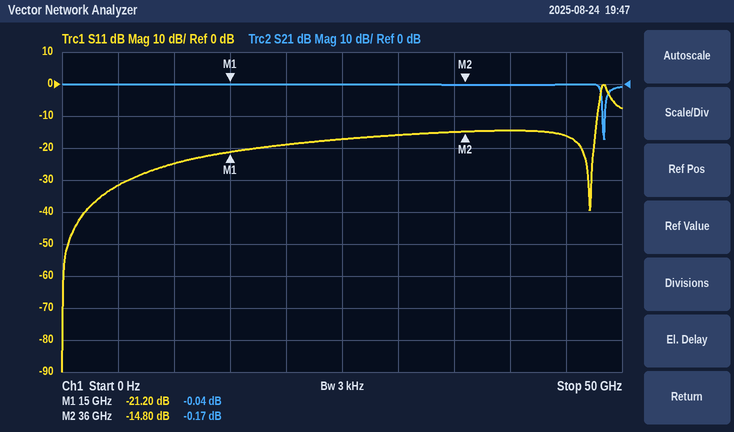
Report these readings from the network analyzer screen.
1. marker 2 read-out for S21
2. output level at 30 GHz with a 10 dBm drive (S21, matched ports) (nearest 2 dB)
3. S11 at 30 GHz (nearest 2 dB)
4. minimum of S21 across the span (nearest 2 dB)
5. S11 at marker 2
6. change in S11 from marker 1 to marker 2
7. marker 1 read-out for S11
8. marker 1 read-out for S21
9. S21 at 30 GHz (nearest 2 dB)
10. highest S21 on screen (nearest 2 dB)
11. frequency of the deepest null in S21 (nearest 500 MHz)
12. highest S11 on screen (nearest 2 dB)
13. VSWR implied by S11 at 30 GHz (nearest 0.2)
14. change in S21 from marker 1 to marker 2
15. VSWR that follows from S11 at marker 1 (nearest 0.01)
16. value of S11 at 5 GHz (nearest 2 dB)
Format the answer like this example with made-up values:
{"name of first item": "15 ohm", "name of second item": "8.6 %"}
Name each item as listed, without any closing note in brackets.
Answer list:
{"marker 2 read-out for S21": "-0.17 dB", "output level at 30 GHz with a 10 dBm drive (S21, matched ports)": "10 dBm", "S11 at 30 GHz": "-16 dB", "minimum of S21 across the span": "-18 dB", "S11 at marker 2": "-14.80 dB", "change in S11 from marker 1 to marker 2": "6.40 dB", "marker 1 read-out for S11": "-21.20 dB", "marker 1 read-out for S21": "-0.04 dB", "S21 at 30 GHz": "0 dB", "highest S21 on screen": "0 dB", "frequency of the deepest null in S21": "48.5 GHz", "highest S11 on screen": "0 dB", "VSWR implied by S11 at 30 GHz": "1.4", "change in S21 from marker 1 to marker 2": "-0.13 dB", "VSWR that follows from S11 at marker 1": "1.19", "value of S11 at 5 GHz": "-32 dB"}
